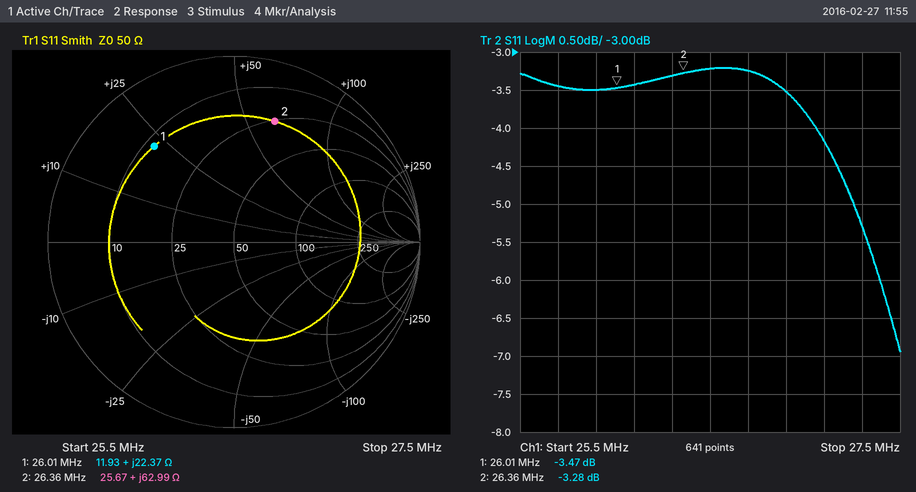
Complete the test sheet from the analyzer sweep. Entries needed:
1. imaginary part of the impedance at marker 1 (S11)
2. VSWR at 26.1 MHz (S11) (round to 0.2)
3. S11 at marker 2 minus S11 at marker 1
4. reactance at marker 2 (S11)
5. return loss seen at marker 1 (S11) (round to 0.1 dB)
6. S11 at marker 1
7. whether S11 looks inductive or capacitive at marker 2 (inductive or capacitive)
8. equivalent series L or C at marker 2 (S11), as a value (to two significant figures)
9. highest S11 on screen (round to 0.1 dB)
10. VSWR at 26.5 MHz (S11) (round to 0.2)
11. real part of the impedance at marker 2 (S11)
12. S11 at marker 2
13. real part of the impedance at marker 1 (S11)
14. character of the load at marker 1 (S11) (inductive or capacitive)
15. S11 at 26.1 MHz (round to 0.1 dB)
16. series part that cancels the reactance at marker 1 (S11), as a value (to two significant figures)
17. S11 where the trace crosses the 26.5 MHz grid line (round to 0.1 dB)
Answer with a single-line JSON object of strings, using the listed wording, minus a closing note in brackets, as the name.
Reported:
{"imaginary part of the impedance at marker 1": "+22.37 Ω", "VSWR at 26.1 MHz (S11)": "5.2", "S11 at marker 2 minus S11 at marker 1": "0.19 dB", "reactance at marker 2": "+62.99 Ω", "return loss seen at marker 1 (S11)": "3.5 dB", "S11 at marker 1": "-3.47 dB", "whether S11 looks inductive or capacitive at marker 2": "inductive", "equivalent series L or C at marker 2 (S11), as a value": "380 nH", "highest S11 on screen": "-3.2 dB", "VSWR at 26.5 MHz (S11)": "5.4", "real part of the impedance at marker 2": "25.67 Ω", "S11 at marker 2": "-3.28 dB", "real part of the impedance at marker 1": "11.93 Ω", "character of the load at marker 1 (S11)": "inductive", "S11 at 26.1 MHz": "-3.4 dB", "series part that cancels the reactance at marker 1 (S11), as a value": "270 pF", "S11 where the trace crosses the 26.5 MHz grid line": "-3.2 dB"}
